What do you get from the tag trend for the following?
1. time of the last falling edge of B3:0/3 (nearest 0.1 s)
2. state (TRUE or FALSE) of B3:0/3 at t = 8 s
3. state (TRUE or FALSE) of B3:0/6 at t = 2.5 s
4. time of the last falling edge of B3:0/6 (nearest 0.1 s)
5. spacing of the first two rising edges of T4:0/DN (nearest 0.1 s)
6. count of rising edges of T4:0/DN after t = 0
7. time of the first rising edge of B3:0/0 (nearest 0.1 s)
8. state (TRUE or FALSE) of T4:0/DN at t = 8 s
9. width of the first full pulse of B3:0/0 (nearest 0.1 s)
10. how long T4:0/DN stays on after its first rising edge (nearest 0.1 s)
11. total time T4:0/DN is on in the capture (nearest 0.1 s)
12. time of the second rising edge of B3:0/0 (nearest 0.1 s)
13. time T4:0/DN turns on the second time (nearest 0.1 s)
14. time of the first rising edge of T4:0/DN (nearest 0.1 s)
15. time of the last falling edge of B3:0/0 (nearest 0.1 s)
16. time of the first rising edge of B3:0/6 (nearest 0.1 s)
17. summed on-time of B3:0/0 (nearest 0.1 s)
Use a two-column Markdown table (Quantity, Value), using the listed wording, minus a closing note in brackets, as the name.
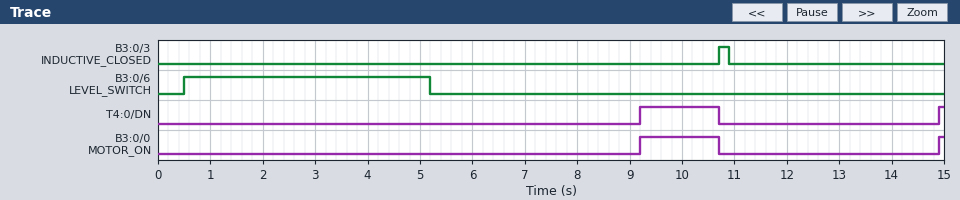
| Quantity | Value |
|---|---|
| time of the last falling edge of B3:0/3 | 10.9 s |
| state (TRUE or FALSE) of B3:0/3 at t = 8 s | FALSE |
| state (TRUE or FALSE) of B3:0/6 at t = 2.5 s | TRUE |
| time of the last falling edge of B3:0/6 | 5.2 s |
| spacing of the first two rising edges of T4:0/DN | 5.7 s |
| count of rising edges of T4:0/DN after t = 0 | 2 |
| time of the first rising edge of B3:0/0 | 9.2 s |
| state (TRUE or FALSE) of T4:0/DN at t = 8 s | FALSE |
| width of the first full pulse of B3:0/0 | 1.5 s |
| how long T4:0/DN stays on after its first rising edge | 1.5 s |
| total time T4:0/DN is on in the capture | 1.6 s |
| time of the second rising edge of B3:0/0 | 14.9 s |
| time T4:0/DN turns on the second time | 14.9 s |
| time of the first rising edge of T4:0/DN | 9.2 s |
| time of the last falling edge of B3:0/0 | 10.7 s |
| time of the first rising edge of B3:0/6 | 0.5 s |
| summed on-time of B3:0/0 | 1.6 s |
